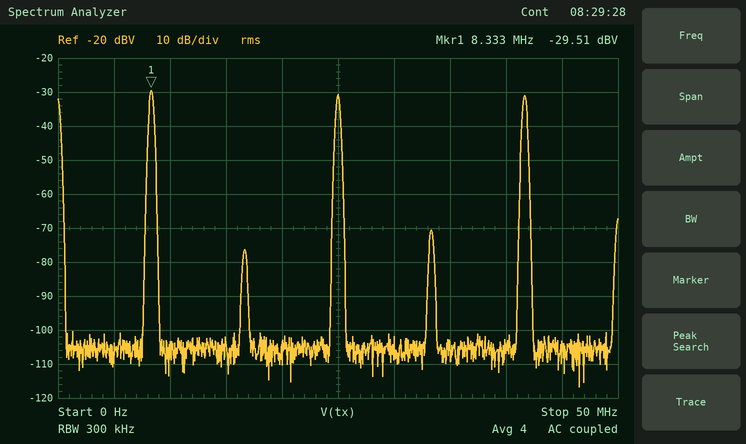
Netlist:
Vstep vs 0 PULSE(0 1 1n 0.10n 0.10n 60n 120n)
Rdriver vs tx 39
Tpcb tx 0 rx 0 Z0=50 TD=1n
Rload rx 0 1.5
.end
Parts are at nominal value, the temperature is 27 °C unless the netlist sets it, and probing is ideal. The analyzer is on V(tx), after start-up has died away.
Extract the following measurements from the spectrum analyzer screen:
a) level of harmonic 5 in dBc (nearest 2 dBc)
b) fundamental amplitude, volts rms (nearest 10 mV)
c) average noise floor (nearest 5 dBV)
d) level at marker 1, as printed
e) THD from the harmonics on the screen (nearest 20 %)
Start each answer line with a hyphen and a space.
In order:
- -2 dBc
- 30 mV
- -105 dBV
- -29.51 dBV
- 120 %
